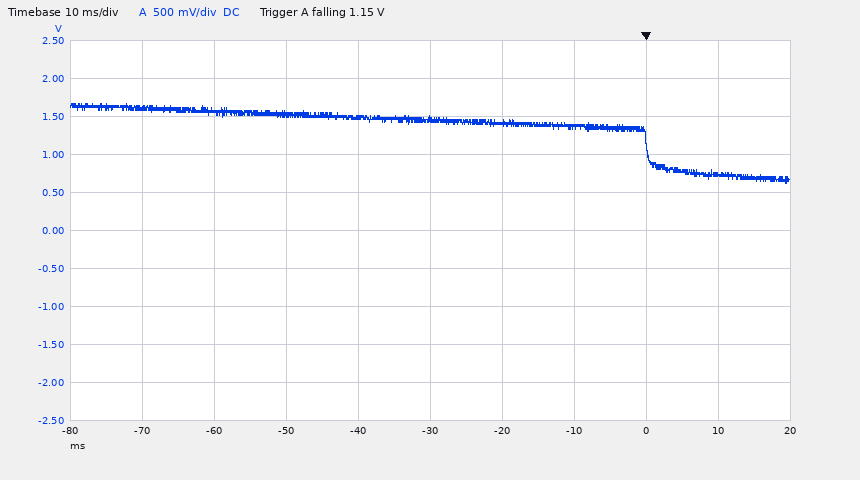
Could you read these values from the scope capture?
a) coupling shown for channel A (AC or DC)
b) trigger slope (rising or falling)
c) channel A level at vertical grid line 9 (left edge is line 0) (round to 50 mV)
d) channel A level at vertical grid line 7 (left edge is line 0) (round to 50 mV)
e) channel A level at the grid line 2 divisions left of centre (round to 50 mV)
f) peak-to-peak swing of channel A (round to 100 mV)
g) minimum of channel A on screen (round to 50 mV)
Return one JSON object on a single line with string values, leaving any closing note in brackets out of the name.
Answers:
{"coupling shown for channel A": "DC", "trigger slope": "falling", "channel A level at vertical grid line 9 (left edge is line 0)": "750 mV", "channel A level at vertical grid line 7 (left edge is line 0)": "1.35 V", "channel A level at the grid line 2 divisions left of centre": "1.55 V", "peak-to-peak swing of channel A": "1.10 V", "minimum of channel A on screen": "600 mV"}
